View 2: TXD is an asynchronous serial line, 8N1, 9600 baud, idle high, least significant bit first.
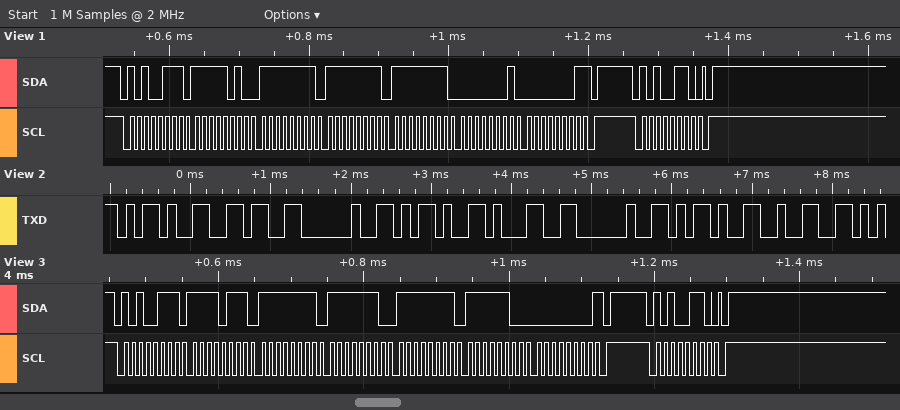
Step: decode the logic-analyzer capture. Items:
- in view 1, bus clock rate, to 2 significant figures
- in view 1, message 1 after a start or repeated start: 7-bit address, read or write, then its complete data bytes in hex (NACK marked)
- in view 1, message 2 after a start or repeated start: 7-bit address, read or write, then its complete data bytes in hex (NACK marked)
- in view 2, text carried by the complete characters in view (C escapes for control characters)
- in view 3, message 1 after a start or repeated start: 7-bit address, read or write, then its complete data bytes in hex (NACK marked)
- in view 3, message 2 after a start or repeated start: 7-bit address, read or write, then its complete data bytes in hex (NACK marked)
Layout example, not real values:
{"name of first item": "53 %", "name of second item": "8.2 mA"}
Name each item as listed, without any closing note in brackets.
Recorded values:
{"in view 1, bus clock rate, to 2 significant figures": "100 kHz", "in view 1, message 1 after a start or repeated start: 7-bit address, read or write, then its complete data bytes in hex": "0x53 read: FA FF FF FF 01 01 NACK", "in view 1, message 2 after a start or repeated start: 7-bit address, read or write, then its complete data bytes in hex": "0x53 write", "in view 2, text carried by the complete characters in view": "\"-6 -1 -2\"", "in view 3, message 1 after a start or repeated start: 7-bit address, read or write, then its complete data bytes in hex": "0x53 read: F7 FF FE FF FC 00 NACK", "in view 3, message 2 after a start or repeated start: 7-bit address, read or write, then its complete data bytes in hex": "0x53 write"}
